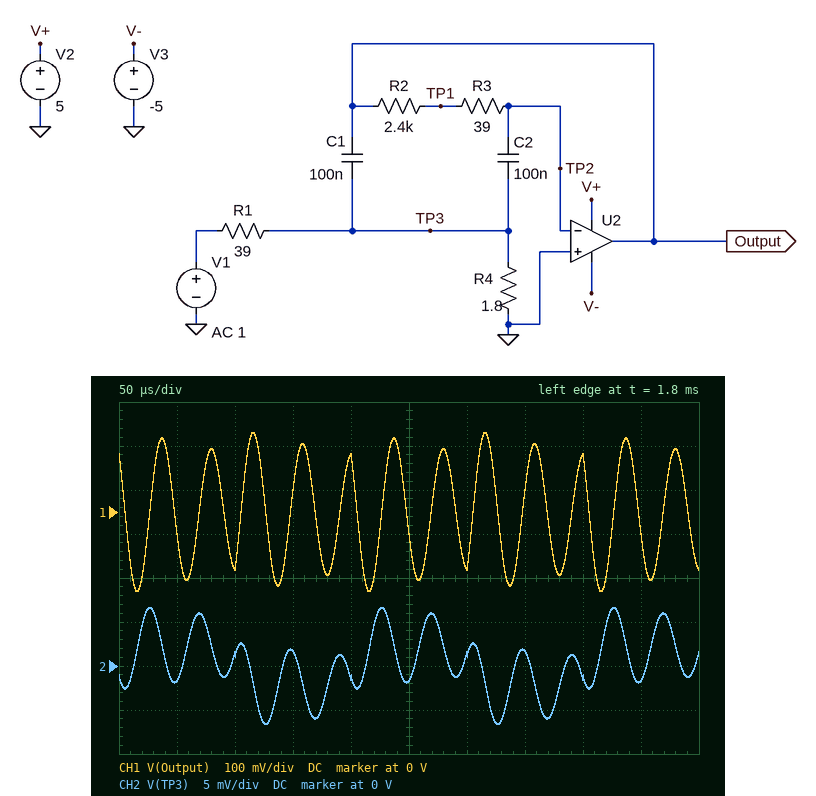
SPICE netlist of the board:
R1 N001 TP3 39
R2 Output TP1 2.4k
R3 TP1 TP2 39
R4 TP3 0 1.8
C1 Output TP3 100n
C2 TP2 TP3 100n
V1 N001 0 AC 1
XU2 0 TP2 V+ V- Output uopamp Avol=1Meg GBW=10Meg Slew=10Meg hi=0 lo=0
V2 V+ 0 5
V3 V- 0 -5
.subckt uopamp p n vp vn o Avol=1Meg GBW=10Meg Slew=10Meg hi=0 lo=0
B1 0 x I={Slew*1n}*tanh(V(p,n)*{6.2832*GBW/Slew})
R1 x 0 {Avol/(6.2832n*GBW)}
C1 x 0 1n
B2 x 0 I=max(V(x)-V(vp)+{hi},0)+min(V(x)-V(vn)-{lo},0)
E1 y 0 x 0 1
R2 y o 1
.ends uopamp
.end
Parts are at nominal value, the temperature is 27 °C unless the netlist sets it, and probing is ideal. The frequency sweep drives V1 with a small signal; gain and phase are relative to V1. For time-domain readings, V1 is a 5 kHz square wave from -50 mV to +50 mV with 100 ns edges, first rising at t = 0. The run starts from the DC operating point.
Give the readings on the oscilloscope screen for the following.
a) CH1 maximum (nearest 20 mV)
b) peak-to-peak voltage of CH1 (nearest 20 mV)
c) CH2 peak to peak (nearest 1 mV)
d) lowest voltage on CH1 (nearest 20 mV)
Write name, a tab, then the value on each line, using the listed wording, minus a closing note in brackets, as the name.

CH1 maximum	180 mV
peak-to-peak voltage of CH1	360 mV
CH2 peak to peak	13 mV
lowest voltage on CH1	-180 mV
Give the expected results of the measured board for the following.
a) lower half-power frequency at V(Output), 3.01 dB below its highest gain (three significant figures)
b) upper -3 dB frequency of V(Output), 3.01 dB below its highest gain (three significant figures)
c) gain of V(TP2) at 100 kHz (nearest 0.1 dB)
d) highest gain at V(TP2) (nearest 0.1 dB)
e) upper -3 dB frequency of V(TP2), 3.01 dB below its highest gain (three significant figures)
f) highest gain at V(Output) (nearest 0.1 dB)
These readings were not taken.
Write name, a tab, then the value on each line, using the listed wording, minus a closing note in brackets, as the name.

lower half-power frequency at V(Output), 3.01 dB below its highest gain	22.9 kHz
upper -3 dB frequency of V(Output), 3.01 dB below its highest gain	24.1 kHz
gain of V(TP2) at 100 kHz	-48.0 dB
highest gain at V(TP2)	-22.5 dB
upper -3 dB frequency of V(TP2), 3.01 dB below its highest gain	24.1 kHz
highest gain at V(Output)	30.1 dB
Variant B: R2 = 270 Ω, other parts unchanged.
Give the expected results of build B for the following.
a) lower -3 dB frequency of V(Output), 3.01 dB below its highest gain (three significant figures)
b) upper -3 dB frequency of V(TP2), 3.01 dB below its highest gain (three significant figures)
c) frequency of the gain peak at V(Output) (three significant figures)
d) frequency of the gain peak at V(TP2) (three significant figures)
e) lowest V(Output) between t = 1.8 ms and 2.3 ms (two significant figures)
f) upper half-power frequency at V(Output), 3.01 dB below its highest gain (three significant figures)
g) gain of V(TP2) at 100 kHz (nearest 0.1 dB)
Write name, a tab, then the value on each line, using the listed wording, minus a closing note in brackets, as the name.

lower -3 dB frequency of V(Output), 3.01 dB below its highest gain	61.6 kHz
upper -3 dB frequency of V(TP2), 3.01 dB below its highest gain	71.6 kHz
frequency of the gain peak at V(Output)	66.0 kHz
frequency of the gain peak at V(TP2)	66.4 kHz
lowest V(Output) between t = 1.8 ms and 2.3 ms	-54 mV
upper half-power frequency at V(Output), 3.01 dB below its highest gain	70.8 kHz
gain of V(TP2) at 100 kHz	-43.6 dB
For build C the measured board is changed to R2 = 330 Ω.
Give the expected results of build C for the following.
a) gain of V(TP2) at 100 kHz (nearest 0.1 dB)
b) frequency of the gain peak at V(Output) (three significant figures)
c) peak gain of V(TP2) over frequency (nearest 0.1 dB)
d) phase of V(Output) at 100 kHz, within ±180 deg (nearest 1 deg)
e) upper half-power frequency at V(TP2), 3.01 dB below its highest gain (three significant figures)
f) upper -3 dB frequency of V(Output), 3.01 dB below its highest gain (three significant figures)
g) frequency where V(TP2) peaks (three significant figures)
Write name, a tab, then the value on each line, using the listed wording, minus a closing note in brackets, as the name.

gain of V(TP2) at 100 kHz	-44.6 dB
frequency of the gain peak at V(Output)	60.4 kHz
peak gain of V(TP2) over frequency	-30.6 dB
phase of V(Output) at 100 kHz, within ±180 deg	96 deg
upper half-power frequency at V(TP2), 3.01 dB below its highest gain	65.0 kHz
upper -3 dB frequency of V(Output), 3.01 dB below its highest gain	64.4 kHz
frequency where V(TP2) peaks	60.7 kHz
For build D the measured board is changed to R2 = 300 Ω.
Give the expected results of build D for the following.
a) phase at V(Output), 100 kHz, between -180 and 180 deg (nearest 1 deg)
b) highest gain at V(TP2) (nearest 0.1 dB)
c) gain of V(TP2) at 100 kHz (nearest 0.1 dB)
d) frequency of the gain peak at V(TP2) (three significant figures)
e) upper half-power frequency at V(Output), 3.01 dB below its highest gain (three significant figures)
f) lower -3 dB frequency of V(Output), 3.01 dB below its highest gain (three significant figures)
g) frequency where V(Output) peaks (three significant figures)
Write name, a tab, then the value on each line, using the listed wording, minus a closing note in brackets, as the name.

phase at V(Output), 100 kHz, between -180 and 180 deg	97 deg
highest gain at V(TP2)	-31.0 dB
gain of V(TP2) at 100 kHz	-44.2 dB
frequency of the gain peak at V(TP2)	63.3 kHz
upper half-power frequency at V(Output), 3.01 dB below its highest gain	67.4 kHz
lower -3 dB frequency of V(Output), 3.01 dB below its highest gain	59.0 kHz
frequency where V(Output) peaks	63.0 kHz
